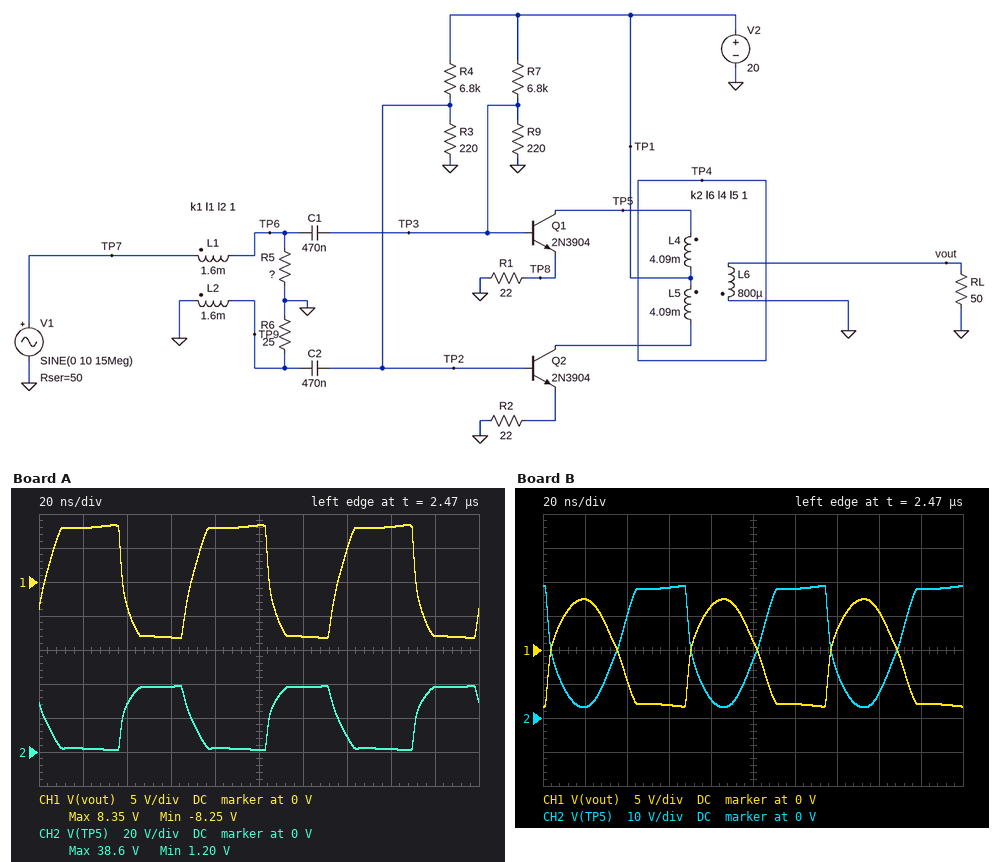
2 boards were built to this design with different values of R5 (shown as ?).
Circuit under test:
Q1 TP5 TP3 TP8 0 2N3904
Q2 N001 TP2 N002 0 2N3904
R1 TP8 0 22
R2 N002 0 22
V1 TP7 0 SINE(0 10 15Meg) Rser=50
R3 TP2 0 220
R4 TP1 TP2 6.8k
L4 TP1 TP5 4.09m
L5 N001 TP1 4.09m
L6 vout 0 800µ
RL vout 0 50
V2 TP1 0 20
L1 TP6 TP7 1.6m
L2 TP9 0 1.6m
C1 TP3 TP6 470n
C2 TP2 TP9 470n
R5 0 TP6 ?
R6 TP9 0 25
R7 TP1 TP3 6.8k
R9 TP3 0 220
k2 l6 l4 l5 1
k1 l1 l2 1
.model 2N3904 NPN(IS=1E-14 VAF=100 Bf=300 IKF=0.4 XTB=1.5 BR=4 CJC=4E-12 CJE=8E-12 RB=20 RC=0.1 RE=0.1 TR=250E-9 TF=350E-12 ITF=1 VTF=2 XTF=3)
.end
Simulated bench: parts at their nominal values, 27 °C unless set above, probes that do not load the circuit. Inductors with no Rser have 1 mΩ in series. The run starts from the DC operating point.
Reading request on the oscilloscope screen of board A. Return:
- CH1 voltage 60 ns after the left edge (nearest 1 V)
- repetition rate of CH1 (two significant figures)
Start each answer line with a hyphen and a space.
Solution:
- -8 V
- 15 MHz
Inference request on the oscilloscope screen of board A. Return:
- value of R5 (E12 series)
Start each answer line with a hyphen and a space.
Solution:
- 33 Ω
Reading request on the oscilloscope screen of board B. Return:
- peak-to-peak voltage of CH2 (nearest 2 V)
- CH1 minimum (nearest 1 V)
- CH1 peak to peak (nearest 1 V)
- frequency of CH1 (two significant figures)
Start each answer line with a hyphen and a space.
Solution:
- 36 V
- -8 V
- 16 V
- 15 MHz
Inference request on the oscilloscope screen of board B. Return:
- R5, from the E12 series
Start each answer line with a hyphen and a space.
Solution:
- 15 Ω
